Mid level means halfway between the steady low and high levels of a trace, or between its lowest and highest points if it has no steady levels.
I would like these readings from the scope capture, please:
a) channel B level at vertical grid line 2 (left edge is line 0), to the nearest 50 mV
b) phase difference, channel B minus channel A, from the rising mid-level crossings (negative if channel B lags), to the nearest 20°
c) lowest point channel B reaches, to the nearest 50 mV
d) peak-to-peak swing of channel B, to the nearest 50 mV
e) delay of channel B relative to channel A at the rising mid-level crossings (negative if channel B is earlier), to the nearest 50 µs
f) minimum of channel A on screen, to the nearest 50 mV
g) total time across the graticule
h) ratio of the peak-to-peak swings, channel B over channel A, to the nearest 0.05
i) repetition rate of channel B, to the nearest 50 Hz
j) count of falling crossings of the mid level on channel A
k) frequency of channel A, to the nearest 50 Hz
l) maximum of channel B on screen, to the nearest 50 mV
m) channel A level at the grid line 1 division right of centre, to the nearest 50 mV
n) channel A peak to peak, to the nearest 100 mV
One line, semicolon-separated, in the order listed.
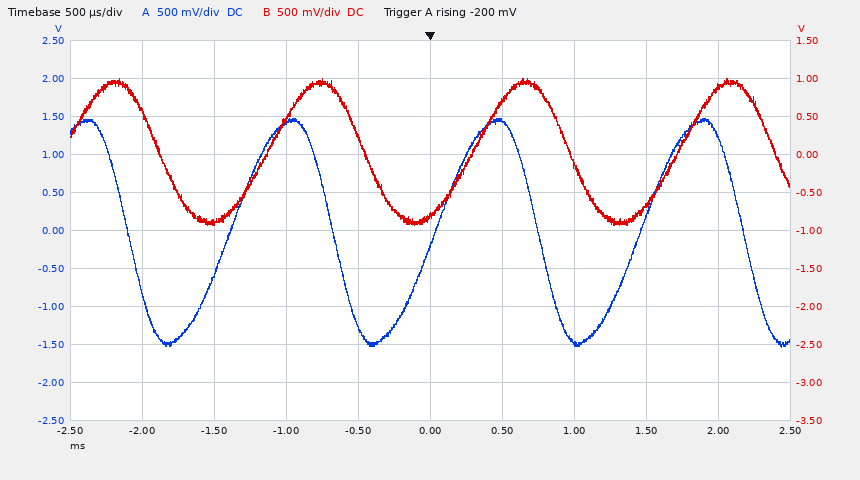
-900 mV; -60°; -950 mV; 1.95 V; +250 µs; -1.55 V; 5 ms; 0.65; 700 Hz; 4; 700 Hz; 1.00 V; 1.45 V; 3.00 V
